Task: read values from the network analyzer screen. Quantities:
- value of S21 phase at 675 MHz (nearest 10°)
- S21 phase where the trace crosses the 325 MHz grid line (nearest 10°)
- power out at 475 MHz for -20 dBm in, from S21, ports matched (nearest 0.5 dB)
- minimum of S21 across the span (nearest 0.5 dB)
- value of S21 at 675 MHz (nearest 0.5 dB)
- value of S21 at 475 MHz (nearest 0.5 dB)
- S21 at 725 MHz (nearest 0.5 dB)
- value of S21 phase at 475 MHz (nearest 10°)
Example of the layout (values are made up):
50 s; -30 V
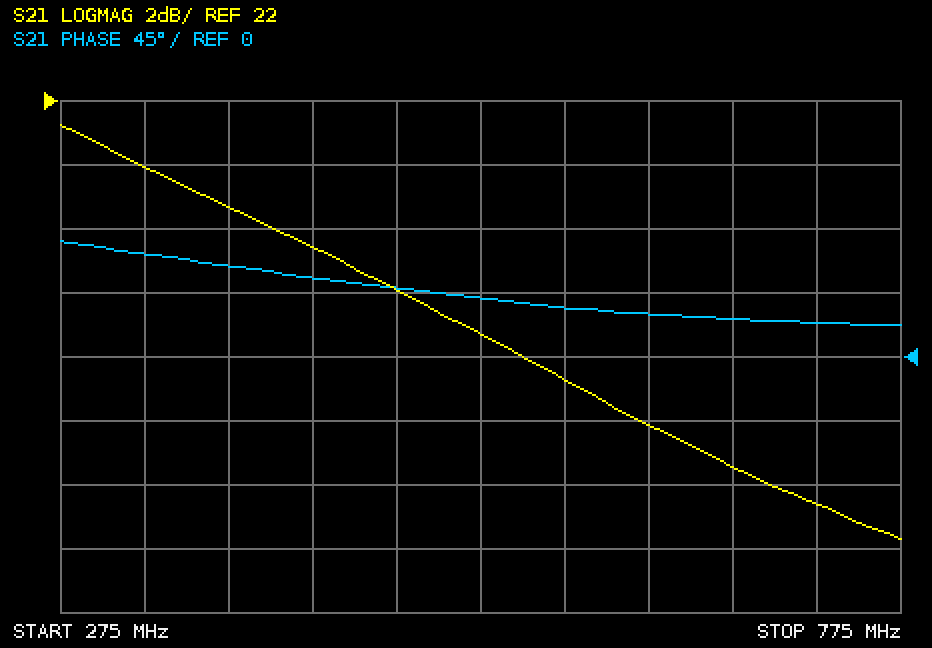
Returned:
30°; 70°; -4.0 dBm; 8.5 dB; 10.5 dB; 16.0 dB; 9.5 dB; 50°
